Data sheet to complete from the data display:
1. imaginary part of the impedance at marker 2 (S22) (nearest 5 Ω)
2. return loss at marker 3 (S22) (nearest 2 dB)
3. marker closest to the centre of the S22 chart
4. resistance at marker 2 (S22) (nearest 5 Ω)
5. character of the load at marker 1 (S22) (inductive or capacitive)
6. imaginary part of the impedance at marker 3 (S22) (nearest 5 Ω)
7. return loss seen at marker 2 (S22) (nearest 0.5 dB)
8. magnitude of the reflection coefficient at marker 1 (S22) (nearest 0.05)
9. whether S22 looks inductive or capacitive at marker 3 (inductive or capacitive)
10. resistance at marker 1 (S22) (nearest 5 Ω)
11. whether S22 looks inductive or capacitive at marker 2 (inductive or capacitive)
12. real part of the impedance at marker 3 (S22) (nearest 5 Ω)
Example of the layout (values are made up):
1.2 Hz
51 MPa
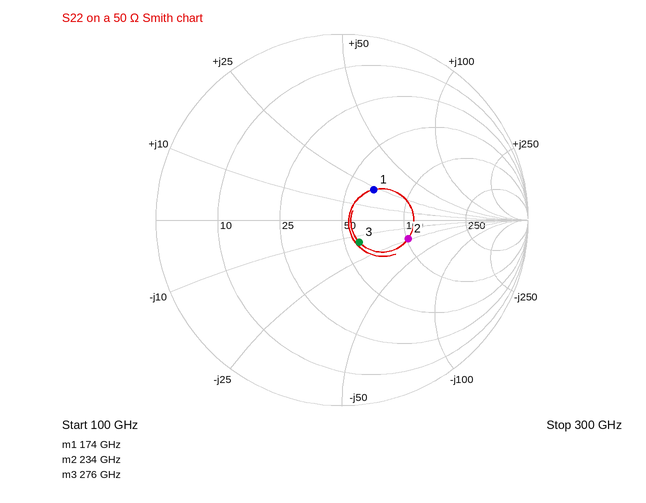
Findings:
-25 Ω
16 dB
marker 3
100 Ω
inductive
-15 Ω
8.5 dB
0.25
capacitive
65 Ω
capacitive
60 Ω
